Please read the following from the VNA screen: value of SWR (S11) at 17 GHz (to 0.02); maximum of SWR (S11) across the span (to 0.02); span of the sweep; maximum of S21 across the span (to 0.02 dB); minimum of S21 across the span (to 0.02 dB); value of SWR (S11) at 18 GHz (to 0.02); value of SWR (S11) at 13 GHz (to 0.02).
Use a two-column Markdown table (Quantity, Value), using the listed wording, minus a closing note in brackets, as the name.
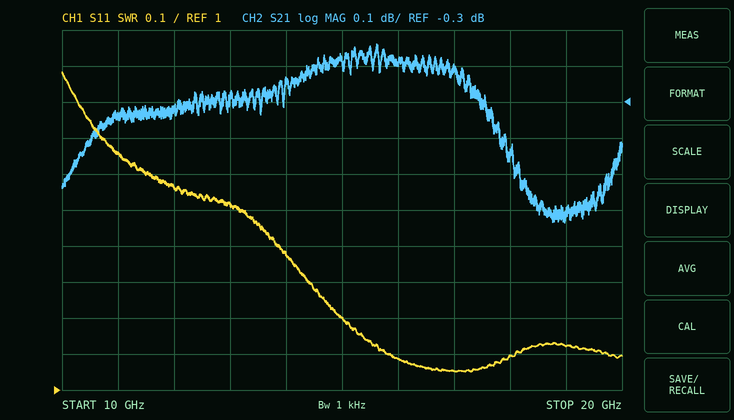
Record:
| Quantity | Value |
|---|---|
| value of SWR (S11) at 17 GHz | 1.06 |
| maximum of SWR (S11) across the span | 1.88 |
| span of the sweep | 10 GHz |
| maximum of S21 across the span | -0.14 dB |
| minimum of S21 across the span | -0.64 dB |
| value of SWR (S11) at 18 GHz | 1.10 |
| value of SWR (S11) at 13 GHz | 1.52 |
